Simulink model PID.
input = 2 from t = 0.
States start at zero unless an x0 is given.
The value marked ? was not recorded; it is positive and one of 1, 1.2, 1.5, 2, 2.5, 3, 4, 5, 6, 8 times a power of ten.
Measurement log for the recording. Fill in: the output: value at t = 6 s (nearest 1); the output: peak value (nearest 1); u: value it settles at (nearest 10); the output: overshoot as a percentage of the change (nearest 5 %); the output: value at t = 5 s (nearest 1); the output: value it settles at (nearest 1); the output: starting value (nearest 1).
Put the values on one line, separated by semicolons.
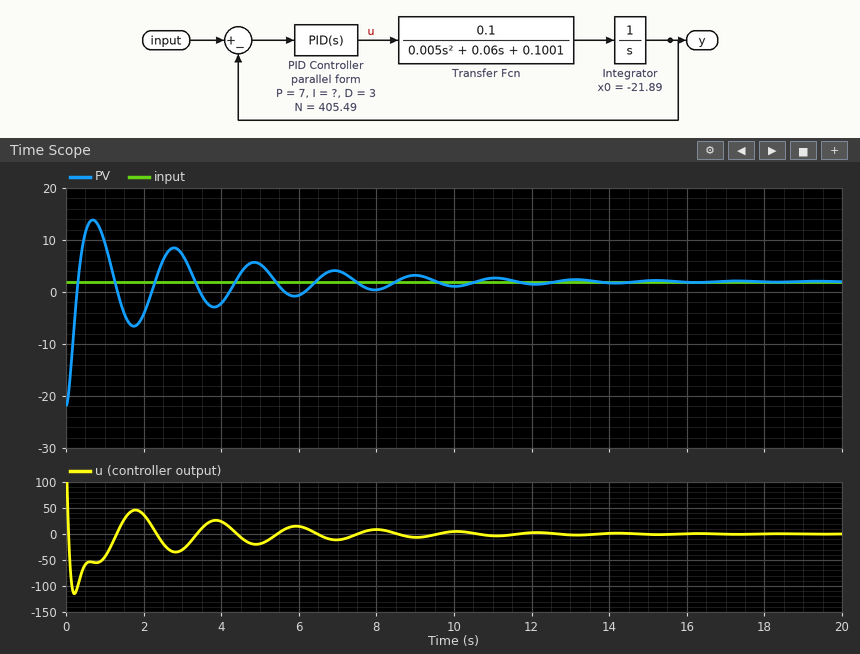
-1; 14; 0; 50 %; 5; 2; -22
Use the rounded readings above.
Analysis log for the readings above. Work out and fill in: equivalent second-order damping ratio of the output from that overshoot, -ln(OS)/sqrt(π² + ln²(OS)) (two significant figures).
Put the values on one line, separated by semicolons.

0.22
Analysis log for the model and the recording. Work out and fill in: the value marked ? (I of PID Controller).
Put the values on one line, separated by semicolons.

30
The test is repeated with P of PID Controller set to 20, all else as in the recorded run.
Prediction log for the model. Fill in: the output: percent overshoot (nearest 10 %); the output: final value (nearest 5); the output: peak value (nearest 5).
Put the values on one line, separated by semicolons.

70 %; 0; 20
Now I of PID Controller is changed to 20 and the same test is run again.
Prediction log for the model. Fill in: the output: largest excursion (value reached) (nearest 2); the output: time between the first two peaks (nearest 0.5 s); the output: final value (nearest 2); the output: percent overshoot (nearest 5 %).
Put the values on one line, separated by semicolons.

10; 2.5 s; 2; 35 %
